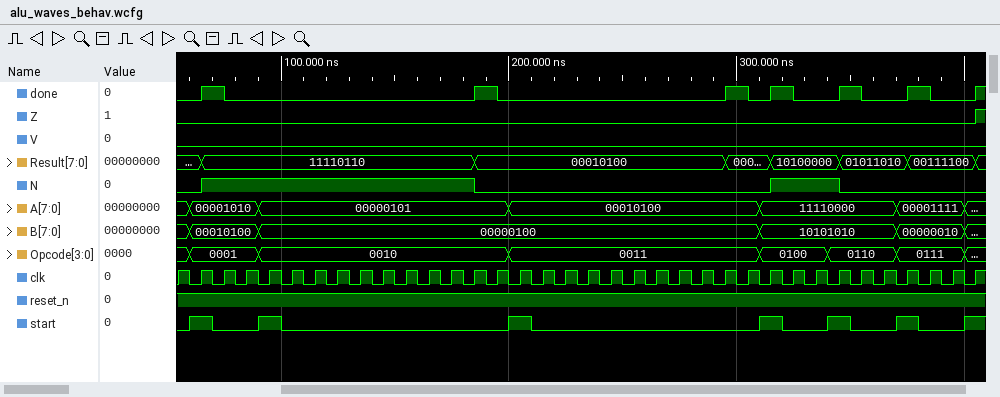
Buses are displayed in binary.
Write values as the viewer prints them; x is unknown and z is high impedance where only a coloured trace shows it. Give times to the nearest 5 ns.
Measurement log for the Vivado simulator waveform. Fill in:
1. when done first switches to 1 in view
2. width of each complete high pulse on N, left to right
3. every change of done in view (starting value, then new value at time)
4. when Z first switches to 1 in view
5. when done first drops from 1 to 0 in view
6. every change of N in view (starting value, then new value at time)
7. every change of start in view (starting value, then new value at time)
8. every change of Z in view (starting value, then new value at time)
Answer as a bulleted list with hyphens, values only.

- 65 ns
- 120 ns, 30 ns
- 0, 1 at 65 ns, 0 at 75 ns, 1 at 185 ns, 0 at 195 ns, 1 at 295 ns, 0 at 305 ns, 1 at 315 ns, 0 at 325 ns, 1 at 345 ns, 0 at 355 ns, 1 at 375 ns, 0 at 385 ns, 1 at 405 ns
- 405 ns
- 75 ns
- 0, 1 at 65 ns, 0 at 185 ns, 1 at 315 ns, 0 at 345 ns
- 0, 1 at 60 ns, 0 at 70 ns, 1 at 90 ns, 0 at 100 ns, 1 at 200 ns, 0 at 210 ns, 1 at 310 ns, 0 at 320 ns, 1 at 340 ns, 0 at 350 ns, 1 at 370 ns, 0 at 380 ns, 1 at 400 ns
- 0, 1 at 405 ns
